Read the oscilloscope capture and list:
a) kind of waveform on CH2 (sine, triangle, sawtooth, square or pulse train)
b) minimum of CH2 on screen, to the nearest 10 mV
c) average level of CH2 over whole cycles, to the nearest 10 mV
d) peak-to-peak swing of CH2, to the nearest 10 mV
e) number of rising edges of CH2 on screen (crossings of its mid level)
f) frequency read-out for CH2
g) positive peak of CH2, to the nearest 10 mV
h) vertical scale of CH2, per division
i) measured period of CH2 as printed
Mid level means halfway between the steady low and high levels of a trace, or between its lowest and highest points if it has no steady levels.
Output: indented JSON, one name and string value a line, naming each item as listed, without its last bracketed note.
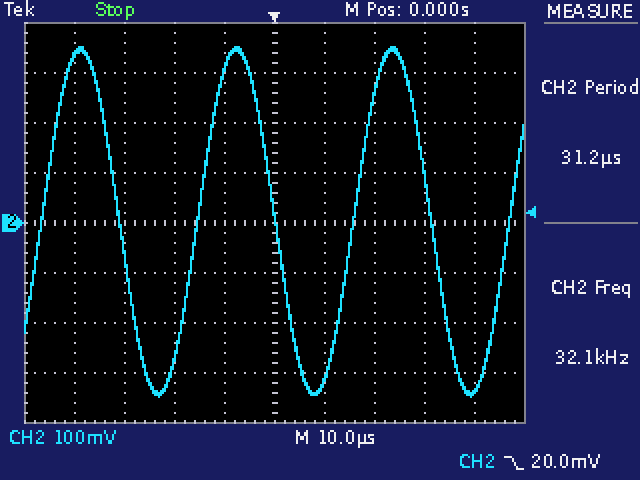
{
  "kind of waveform on CH2": "sine",
  "minimum of CH2 on screen, to the nearest 10 mV": "-350 mV",
  "average level of CH2 over whole cycles, to the nearest 10 mV": "0 mV",
  "peak-to-peak swing of CH2, to the nearest 10 mV": "700 mV",
  "number of rising edges of CH2 on screen": "4",
  "frequency read-out for CH2": "32.1 kHz",
  "positive peak of CH2, to the nearest 10 mV": "350 mV",
  "vertical scale of CH2, per division": "100 mV",
  "measured period of CH2 as printed": "31.2 µs"
}
